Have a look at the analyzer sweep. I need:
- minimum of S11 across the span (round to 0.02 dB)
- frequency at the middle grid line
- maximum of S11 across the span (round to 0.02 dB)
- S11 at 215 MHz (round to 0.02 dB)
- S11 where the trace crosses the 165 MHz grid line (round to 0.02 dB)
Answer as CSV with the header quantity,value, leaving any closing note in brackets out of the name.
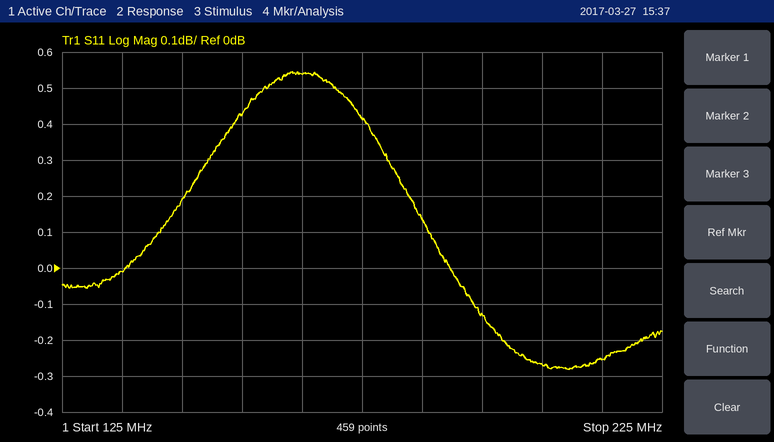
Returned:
quantity,value
minimum of S11 across the span,-0.28 dB
frequency at the middle grid line,175 MHz
maximum of S11 across the span,0.54 dB
S11 at 215 MHz,-0.26 dB
S11 where the trace crosses the 165 MHz grid line,0.54 dB
